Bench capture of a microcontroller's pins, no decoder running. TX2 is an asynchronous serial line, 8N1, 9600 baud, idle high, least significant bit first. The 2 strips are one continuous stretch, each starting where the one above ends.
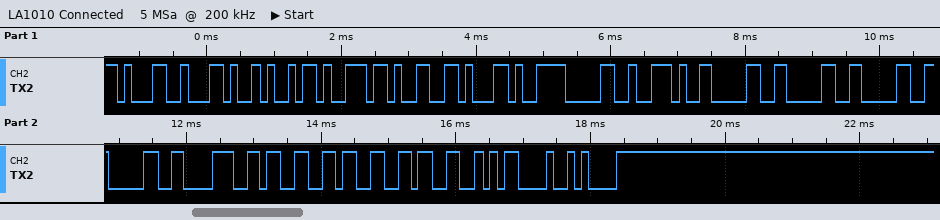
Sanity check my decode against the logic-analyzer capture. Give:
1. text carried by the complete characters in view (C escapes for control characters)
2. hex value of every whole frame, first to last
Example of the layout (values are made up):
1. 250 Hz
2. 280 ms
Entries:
1. "1,inf,0.00008333\r\n"
2. 0x31 0x2C 0x69 0x6E 0x66 0x2C 0x30 0x2E 0x30 0x30 0x30 0x30 0x38 0x33 0x33 0x33 0x0D 0x0A
